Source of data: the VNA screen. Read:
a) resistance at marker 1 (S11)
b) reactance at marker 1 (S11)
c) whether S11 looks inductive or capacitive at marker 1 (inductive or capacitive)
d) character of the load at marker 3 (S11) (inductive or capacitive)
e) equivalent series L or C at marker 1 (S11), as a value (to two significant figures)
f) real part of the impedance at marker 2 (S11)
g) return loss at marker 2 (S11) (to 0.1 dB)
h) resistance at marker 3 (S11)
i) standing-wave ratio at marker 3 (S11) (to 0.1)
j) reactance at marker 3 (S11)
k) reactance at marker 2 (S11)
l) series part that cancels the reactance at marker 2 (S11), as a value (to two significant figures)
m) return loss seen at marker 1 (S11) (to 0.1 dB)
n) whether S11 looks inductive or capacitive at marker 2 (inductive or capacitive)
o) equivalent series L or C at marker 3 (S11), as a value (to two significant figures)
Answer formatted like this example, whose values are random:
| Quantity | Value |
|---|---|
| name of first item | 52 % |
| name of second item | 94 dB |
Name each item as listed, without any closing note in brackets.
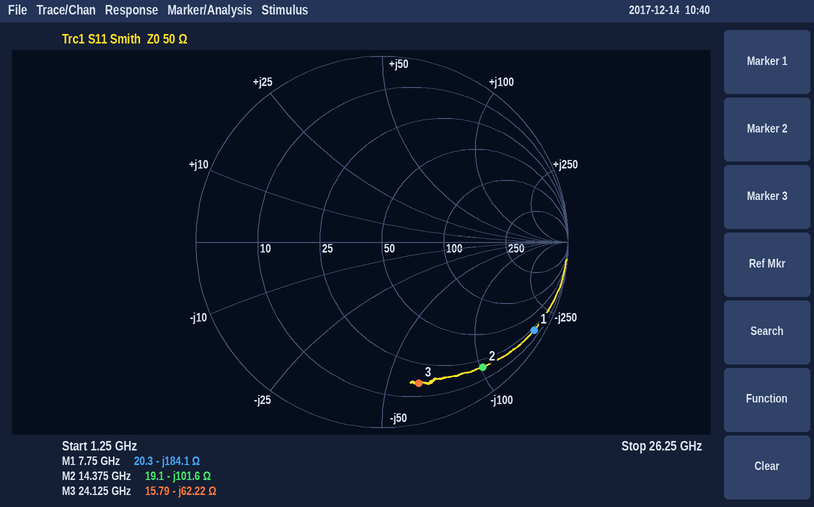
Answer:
| Quantity | Value |
|---|---|
| resistance at marker 1 | 20.3 Ω |
| reactance at marker 1 | -184.1 Ω |
| whether S11 looks inductive or capacitive at marker 1 | capacitive |
| character of the load at marker 3 (S11) | capacitive |
| equivalent series L or C at marker 1 (S11), as a value | 110 fF |
| real part of the impedance at marker 2 | 19.1 Ω |
| return loss at marker 2 (S11) | 1.3 dB |
| resistance at marker 3 | 15.79 Ω |
| standing-wave ratio at marker 3 (S11) | 8.3 |
| reactance at marker 3 | -62.22 Ω |
| reactance at marker 2 | -101.6 Ω |
| series part that cancels the reactance at marker 2 (S11), as a value | 1.1 nH |
| return loss seen at marker 1 (S11) | 0.5 dB |
| whether S11 looks inductive or capacitive at marker 2 | capacitive |
| equivalent series L or C at marker 3 (S11), as a value | 110 fF |
